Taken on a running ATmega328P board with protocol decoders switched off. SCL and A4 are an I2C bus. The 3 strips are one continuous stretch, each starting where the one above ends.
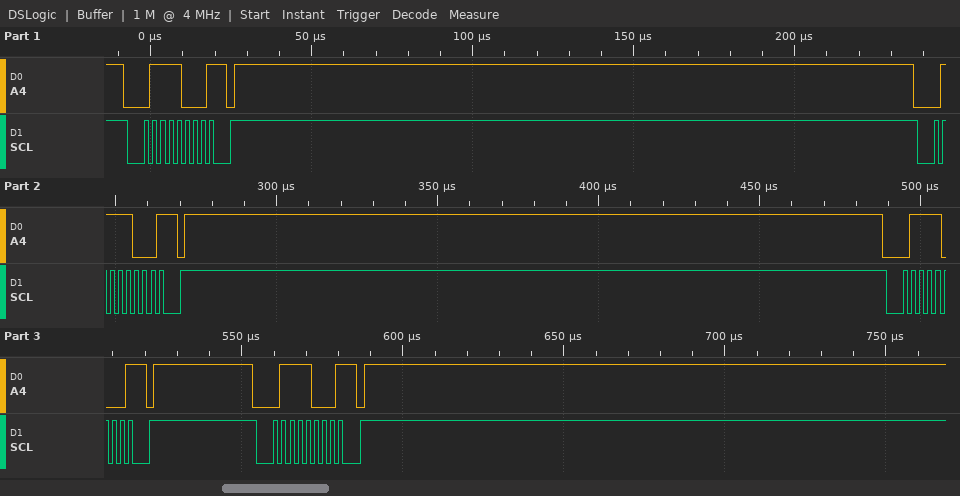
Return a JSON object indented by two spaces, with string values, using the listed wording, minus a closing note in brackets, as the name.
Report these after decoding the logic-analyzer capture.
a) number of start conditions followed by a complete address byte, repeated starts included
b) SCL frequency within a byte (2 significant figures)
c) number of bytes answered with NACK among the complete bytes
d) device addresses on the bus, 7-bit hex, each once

{
  "number of start conditions followed by a complete address byte, repeated starts included": "4",
  "SCL frequency within a byte": "400 kHz",
  "number of bytes answered with NACK among the complete bytes": "4",
  "device addresses on the bus, 7-bit hex, each once": "0x3C"
}
